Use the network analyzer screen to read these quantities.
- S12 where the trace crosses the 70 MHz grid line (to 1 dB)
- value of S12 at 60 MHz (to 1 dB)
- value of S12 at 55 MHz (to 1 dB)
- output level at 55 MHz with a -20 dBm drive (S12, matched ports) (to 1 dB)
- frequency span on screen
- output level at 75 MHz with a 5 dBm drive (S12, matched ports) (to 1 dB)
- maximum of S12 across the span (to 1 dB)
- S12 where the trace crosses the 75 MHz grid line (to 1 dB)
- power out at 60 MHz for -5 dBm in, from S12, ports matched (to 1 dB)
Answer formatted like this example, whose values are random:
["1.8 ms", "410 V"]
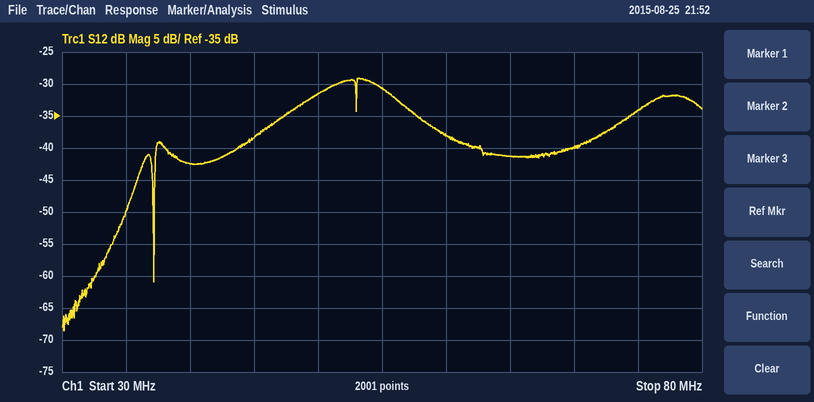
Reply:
["-40 dB", "-38 dB", "-31 dB", "-51 dBm", "50 MHz", "-29 dBm", "-29 dB", "-34 dB", "-43 dBm"]
